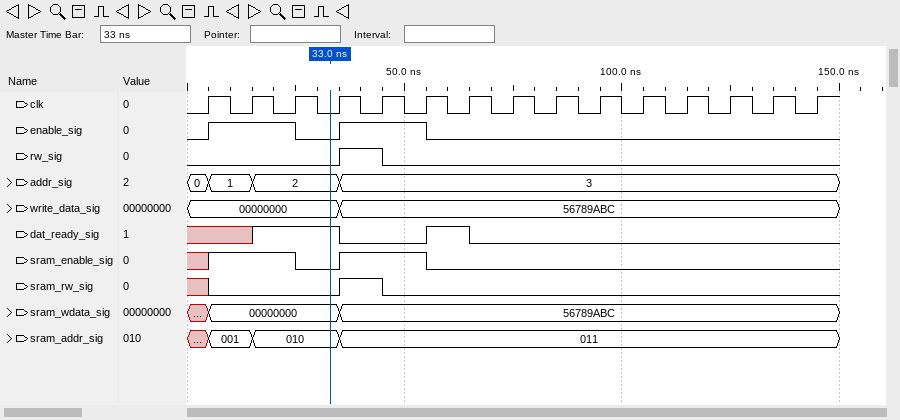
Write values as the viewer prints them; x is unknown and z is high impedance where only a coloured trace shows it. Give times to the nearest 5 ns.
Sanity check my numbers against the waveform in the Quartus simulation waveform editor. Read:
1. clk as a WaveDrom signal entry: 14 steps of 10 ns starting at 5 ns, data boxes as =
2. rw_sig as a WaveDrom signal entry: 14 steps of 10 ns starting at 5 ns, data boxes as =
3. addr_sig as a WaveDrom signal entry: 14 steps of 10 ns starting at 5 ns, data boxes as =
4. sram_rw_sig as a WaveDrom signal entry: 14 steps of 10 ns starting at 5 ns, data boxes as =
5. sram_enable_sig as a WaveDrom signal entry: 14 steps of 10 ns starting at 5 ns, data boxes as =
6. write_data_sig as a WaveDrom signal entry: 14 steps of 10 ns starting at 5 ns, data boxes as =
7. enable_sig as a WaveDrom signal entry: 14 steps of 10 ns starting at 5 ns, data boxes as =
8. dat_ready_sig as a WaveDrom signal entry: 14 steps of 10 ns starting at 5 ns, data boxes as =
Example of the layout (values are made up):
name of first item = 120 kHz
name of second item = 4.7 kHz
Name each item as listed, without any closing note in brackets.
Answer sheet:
clk as a WaveDrom signal entry: 14 steps of 10 ns starting at 5 ns, data boxes as = = {name: 'clk', wave: 'p.............'}
rw_sig as a WaveDrom signal entry: 14 steps of 10 ns starting at 5 ns, data boxes as = = {name: 'rw_sig', wave: '0..10.........'}
addr_sig as a WaveDrom signal entry: 14 steps of 10 ns starting at 5 ns, data boxes as = = {name: 'addr_sig', wave: '==.=..........', data: '1 2 3'}
sram_rw_sig as a WaveDrom signal entry: 14 steps of 10 ns starting at 5 ns, data boxes as = = {name: 'sram_rw_sig', wave: '0..10.........'}
sram_enable_sig as a WaveDrom signal entry: 14 steps of 10 ns starting at 5 ns, data boxes as = = {name: 'sram_enable_sig', wave: '1.01.0........'}
write_data_sig as a WaveDrom signal entry: 14 steps of 10 ns starting at 5 ns, data boxes as = = {name: 'write_data_sig', wave: '=..=..........', data: '00000000 56789ABC'}
enable_sig as a WaveDrom signal entry: 14 steps of 10 ns starting at 5 ns, data boxes as = = {name: 'enable_sig', wave: '1.01.0........'}
dat_ready_sig as a WaveDrom signal entry: 14 steps of 10 ns starting at 5 ns, data boxes as = = {name: 'dat_ready_sig', wave: 'x1.0.10.......'}
